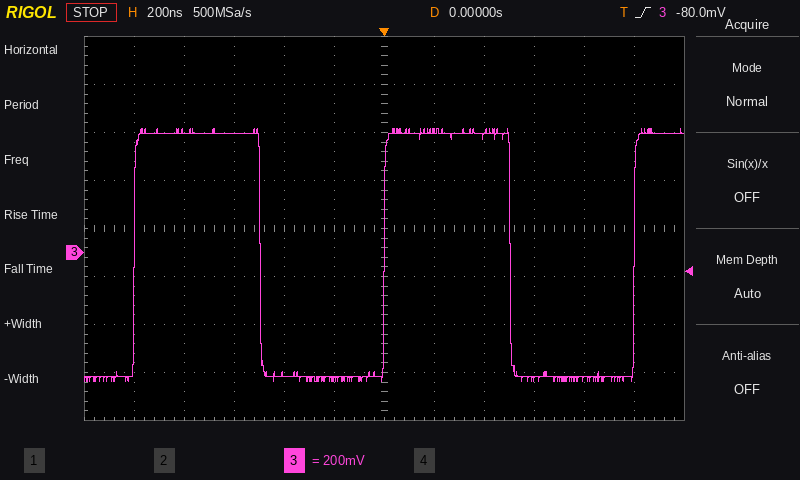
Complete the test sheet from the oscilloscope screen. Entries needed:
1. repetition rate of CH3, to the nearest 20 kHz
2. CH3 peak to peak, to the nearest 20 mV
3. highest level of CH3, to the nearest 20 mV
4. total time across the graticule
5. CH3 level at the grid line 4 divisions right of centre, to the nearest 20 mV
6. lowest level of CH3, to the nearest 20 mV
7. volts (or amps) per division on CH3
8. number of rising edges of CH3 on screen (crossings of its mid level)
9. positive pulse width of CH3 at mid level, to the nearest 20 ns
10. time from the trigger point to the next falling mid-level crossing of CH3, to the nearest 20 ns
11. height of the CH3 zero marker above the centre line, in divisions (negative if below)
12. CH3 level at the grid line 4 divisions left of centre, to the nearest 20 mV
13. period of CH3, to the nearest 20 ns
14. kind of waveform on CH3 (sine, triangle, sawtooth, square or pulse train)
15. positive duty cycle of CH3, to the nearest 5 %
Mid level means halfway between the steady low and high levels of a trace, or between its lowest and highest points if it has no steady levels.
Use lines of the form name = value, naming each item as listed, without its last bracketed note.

repetition rate of CH3, to the nearest 20 kHz = 1.00 MHz
CH3 peak to peak, to the nearest 20 mV = 1.06 V
highest level of CH3, to the nearest 20 mV = 520 mV
total time across the graticule = 2.4 µs
CH3 level at the grid line 4 divisions right of centre, to the nearest 20 mV = -520 mV
lowest level of CH3, to the nearest 20 mV = -540 mV
volts (or amps) per division on CH3 = 200 mV
number of rising edges of CH3 on screen = 3
positive pulse width of CH3 at mid level, to the nearest 20 ns = 500 ns
time from the trigger point to the next falling mid-level crossing of CH3, to the nearest 20 ns = 500 ns
height of the CH3 zero marker above the centre line, in divisions = -0.5 div
CH3 level at the grid line 4 divisions left of centre, to the nearest 20 mV = 500 mV
period of CH3, to the nearest 20 ns = 1.00 µs
kind of waveform on CH3 = square
positive duty cycle of CH3, to the nearest 5 % = 50 %
